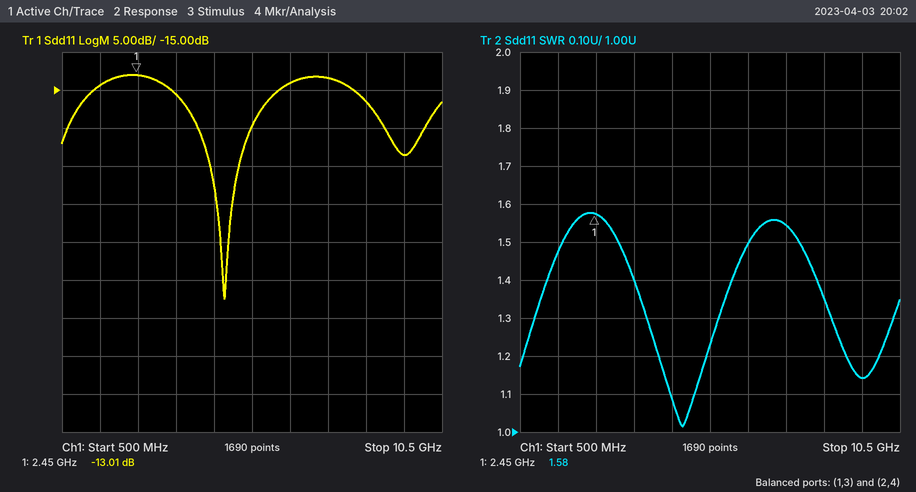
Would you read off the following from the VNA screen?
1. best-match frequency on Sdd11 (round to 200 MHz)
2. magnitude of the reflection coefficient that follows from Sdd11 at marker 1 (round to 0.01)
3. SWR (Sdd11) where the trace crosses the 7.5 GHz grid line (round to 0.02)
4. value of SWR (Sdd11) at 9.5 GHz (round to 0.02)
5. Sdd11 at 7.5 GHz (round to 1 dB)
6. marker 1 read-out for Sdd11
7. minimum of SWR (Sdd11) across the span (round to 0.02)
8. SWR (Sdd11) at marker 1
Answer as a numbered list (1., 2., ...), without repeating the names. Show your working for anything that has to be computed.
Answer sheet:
1. 4.8 GHz
2. 10^(-13.01/20) ≈ 0.22
3. 1.54
4. 1.14
5. -13 dB
6. -13.01 dB
7. 1.02
8. 1.58
